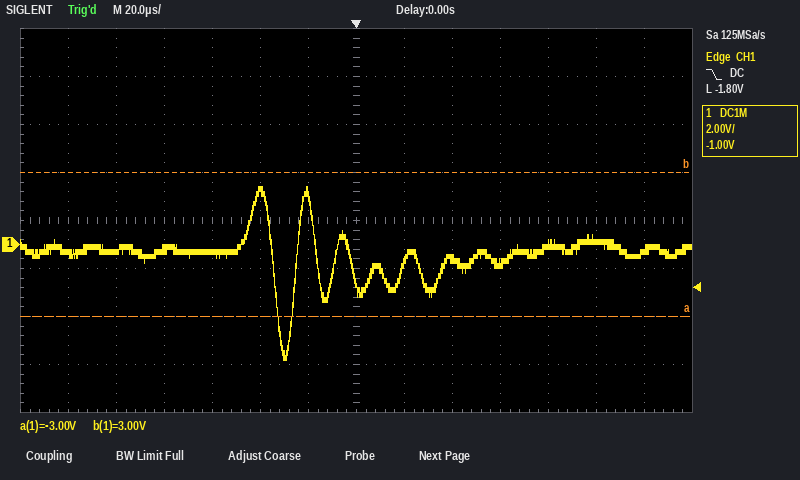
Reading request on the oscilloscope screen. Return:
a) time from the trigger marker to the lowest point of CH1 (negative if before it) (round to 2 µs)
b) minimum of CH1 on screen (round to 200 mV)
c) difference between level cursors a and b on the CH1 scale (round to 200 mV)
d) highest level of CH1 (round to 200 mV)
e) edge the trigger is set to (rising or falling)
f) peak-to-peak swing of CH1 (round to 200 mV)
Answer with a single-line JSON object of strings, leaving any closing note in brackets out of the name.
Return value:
{"time from the trigger marker to the lowest point of CH1 (negative if before it)": "-30 µs", "minimum of CH1 on screen": "-4.8 V", "difference between level cursors a and b on the CH1 scale": "6.0 V", "highest level of CH1": "2.4 V", "edge the trigger is set to": "falling", "peak-to-peak swing of CH1": "7.2 V"}
